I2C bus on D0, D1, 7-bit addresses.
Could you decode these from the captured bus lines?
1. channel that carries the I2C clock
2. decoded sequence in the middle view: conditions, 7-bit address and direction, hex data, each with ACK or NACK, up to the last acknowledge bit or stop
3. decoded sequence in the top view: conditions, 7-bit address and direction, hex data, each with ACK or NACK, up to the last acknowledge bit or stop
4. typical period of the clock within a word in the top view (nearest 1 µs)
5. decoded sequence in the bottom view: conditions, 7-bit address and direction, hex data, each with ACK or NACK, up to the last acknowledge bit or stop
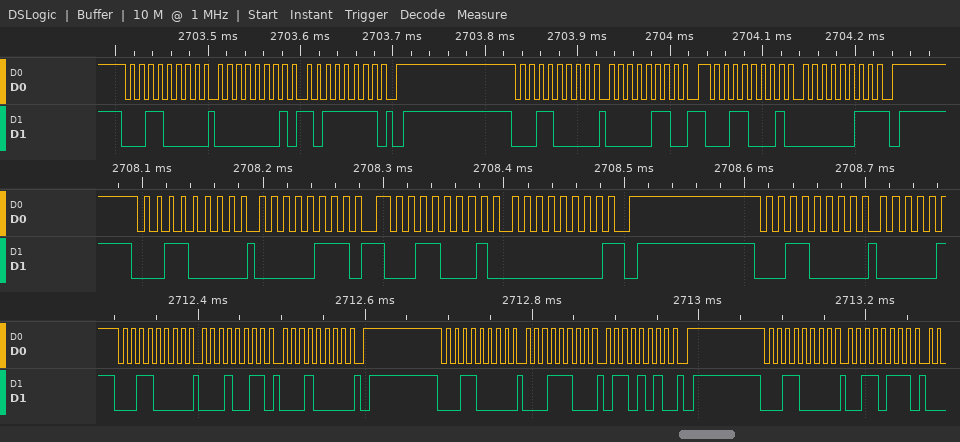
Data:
D0
start, address 18 write ACK, 07 ACK, repeated start, address 18 read ACK, 00 NACK, stop, start, address 18 write ACK
start, address 18 write ACK, 01 ACK, BF ACK, stop, start, address 18 write ACK, 06 ACK, repeated start, address 18 read ACK, 03 NACK, stop
10 µs
start, address 18 write ACK, 13 ACK, 10 ACK, stop, start, address 18 write ACK, 1C ACK, 6A ACK, stop, start, address 18 write ACK, 37 ACK
